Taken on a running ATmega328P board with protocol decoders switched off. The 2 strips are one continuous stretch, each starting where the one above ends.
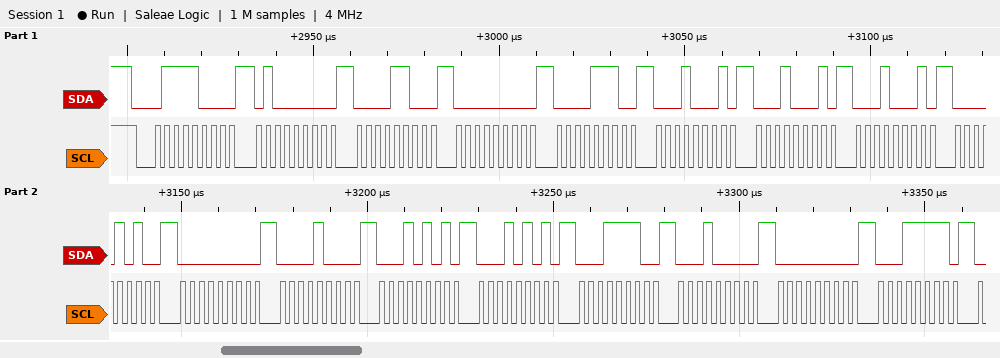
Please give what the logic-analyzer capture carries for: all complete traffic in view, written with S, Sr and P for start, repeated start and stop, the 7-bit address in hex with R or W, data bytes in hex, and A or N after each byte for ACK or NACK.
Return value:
S 3CW A 40 A 0C A 00 A 0E A 11 A 11 A 11 A 0A A 00 A 08 A 15 A 15 A 1E A 10 A 00 A 1F A
